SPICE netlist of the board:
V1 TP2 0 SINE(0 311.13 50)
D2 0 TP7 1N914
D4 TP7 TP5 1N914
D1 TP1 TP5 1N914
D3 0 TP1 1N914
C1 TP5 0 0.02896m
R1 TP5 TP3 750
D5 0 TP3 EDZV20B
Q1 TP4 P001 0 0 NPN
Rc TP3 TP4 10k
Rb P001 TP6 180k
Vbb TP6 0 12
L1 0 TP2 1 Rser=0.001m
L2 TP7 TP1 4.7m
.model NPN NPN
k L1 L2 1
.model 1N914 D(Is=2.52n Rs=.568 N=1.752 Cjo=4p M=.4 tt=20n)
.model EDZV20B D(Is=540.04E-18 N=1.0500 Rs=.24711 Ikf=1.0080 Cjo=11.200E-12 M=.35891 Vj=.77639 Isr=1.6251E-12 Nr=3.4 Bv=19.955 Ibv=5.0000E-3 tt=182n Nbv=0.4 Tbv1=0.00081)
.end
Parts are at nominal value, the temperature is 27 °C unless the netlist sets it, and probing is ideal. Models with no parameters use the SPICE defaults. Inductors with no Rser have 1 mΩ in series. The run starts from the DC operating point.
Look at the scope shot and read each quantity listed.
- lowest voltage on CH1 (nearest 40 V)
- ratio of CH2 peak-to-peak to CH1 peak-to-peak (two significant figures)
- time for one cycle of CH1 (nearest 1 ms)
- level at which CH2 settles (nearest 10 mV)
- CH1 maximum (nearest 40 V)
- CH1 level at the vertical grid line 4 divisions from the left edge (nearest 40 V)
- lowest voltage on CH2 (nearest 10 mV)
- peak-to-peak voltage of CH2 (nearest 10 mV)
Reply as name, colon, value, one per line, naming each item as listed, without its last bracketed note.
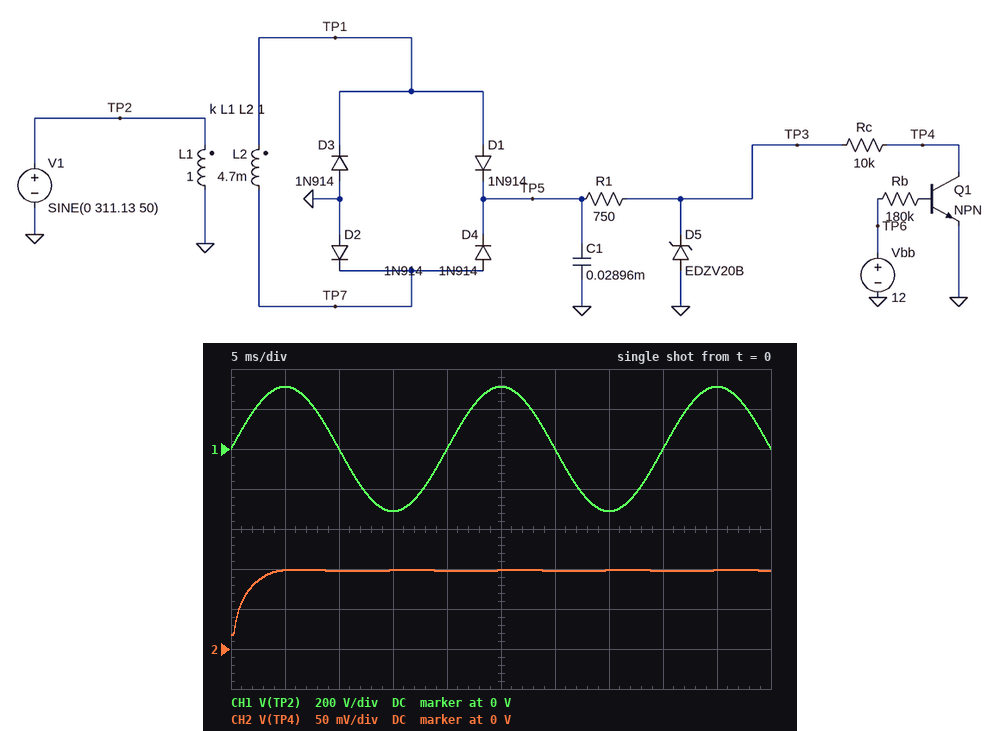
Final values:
lowest voltage on CH1: -320 V
ratio of CH2 peak-to-peak to CH1 peak-to-peak: 0.00013
time for one cycle of CH1: 20 ms
level at which CH2 settles: 100 mV
CH1 maximum: 320 V
CH1 level at the vertical grid line 4 divisions from the left edge: 0 V
lowest voltage on CH2: 20 mV
peak-to-peak voltage of CH2: 80 mV
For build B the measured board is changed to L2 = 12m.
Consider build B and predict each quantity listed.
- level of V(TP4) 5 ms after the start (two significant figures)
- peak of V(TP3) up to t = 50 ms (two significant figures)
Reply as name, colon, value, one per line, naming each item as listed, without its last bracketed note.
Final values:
level of V(TP4) 5 ms after the start: 100 mV
peak of V(TP3) up to t = 50 ms: 20 V
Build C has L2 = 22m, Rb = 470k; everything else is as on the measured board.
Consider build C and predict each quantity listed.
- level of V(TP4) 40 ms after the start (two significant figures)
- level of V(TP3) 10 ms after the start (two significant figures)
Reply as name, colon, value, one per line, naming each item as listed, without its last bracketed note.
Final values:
level of V(TP4) 40 ms after the start: 160 mV
level of V(TP3) 10 ms after the start: 20 V
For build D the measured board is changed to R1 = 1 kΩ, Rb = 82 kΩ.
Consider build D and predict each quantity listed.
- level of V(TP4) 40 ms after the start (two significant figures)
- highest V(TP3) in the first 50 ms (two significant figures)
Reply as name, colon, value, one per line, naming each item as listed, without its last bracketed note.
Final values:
level of V(TP4) 40 ms after the start: 74 mV
highest V(TP3) in the first 50 ms: 18 V
